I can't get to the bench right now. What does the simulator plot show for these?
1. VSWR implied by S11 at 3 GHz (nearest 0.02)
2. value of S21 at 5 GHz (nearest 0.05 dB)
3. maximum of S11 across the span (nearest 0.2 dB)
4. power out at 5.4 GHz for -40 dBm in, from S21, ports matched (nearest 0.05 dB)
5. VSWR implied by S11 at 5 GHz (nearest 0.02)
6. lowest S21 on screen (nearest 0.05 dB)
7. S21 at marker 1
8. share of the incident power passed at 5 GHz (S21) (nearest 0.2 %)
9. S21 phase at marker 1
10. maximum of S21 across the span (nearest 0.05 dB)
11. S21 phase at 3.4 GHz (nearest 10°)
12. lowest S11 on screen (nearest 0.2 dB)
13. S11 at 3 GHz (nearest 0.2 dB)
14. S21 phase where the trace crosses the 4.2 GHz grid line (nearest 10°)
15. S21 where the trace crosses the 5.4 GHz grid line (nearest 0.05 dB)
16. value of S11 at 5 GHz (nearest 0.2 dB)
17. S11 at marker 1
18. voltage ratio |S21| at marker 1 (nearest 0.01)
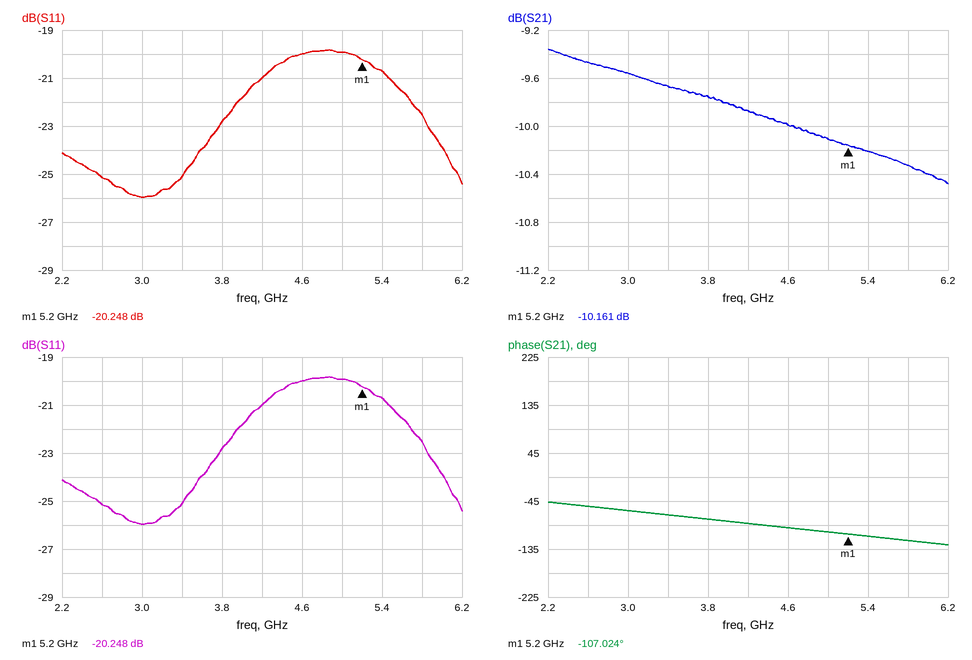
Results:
1.10
-10.10 dB
-19.8 dB
-50.20 dBm
1.22
-10.50 dB
-10.161 dB
9.8 %
-107.024°
-9.35 dB
-70°
-26.0 dB
-26.0 dB
-90°
-10.20 dB
-20.0 dB
-20.248 dB
0.31
